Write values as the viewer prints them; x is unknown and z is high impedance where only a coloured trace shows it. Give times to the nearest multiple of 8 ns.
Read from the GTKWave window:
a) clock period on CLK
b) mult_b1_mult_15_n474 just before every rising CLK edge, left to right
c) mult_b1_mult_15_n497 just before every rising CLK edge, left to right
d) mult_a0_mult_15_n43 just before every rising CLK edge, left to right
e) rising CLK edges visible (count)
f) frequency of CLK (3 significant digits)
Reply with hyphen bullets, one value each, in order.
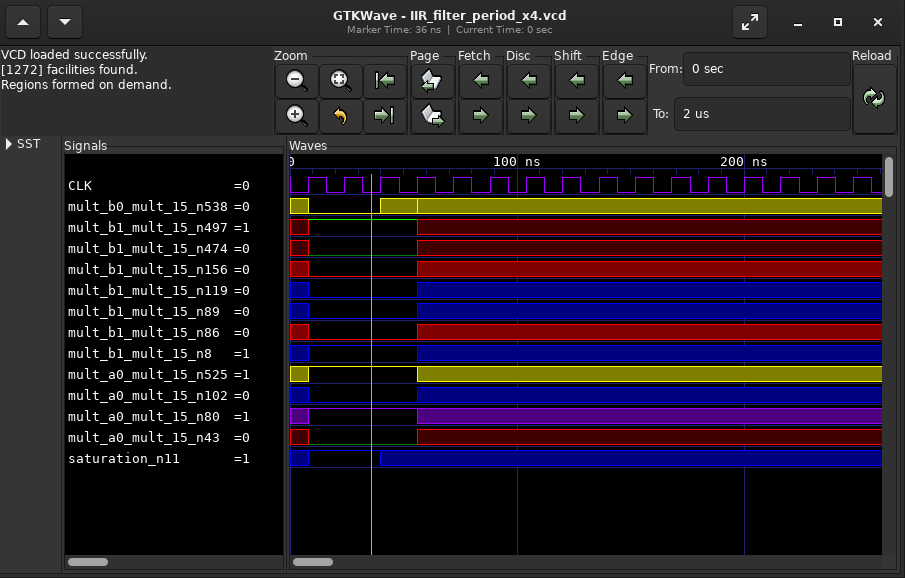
- 16 ns
- x 0 0 0 x x x x x x x x x x x x
- x 1 1 1 x x x x x x x x x x x x
- x 0 0 0 x x x x x x x x x x x x
- 16
- 62.5 MHz
